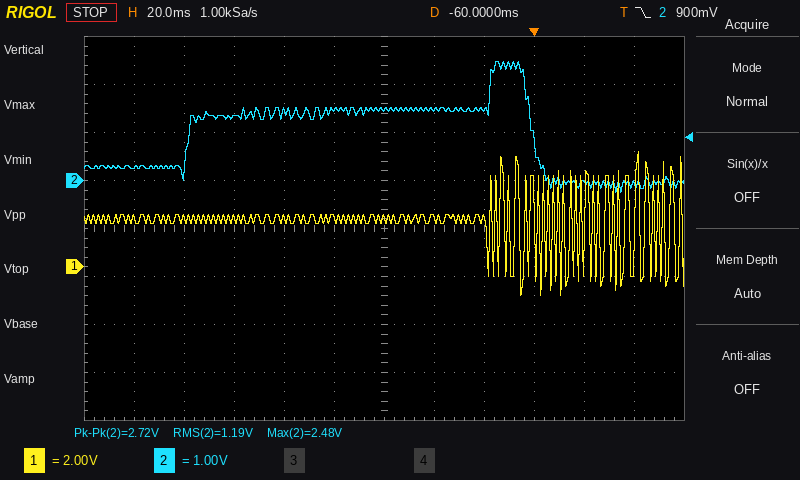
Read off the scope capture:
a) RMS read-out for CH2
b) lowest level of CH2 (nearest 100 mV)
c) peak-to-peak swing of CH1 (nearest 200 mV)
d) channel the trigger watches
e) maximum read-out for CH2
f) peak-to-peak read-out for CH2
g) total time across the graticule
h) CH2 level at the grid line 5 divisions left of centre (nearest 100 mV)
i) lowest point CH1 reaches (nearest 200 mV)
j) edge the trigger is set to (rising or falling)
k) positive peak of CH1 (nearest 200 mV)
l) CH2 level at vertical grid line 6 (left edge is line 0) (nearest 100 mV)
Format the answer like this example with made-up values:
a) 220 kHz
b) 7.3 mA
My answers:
a) 1.19 V
b) -200 mV
c) 6.0 V
d) CH2
e) 2.48 V
f) 2.72 V
g) 240 ms
h) 300 mV
i) -1.2 V
j) falling
k) 4.8 V
l) 1.5 V
